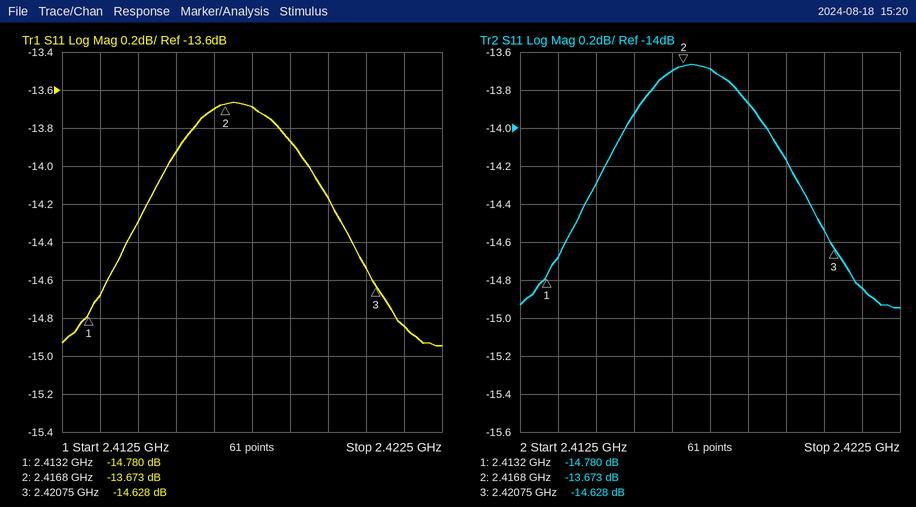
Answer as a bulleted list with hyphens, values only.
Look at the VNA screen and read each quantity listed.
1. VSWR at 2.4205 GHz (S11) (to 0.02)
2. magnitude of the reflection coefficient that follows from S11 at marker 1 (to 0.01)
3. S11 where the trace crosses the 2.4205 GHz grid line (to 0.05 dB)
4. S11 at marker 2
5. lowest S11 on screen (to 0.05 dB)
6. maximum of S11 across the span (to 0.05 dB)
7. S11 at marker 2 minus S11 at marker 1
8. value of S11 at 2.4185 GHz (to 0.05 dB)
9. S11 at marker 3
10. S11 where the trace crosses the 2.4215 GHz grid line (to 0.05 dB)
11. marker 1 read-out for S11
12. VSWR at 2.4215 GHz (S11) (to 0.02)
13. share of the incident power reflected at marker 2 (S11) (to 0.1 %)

- 1.46
- 0.18
- -14.55 dB
- -13.673 dB
- -14.95 dB
- -13.65 dB
- 1.107 dB
- -13.85 dB
- -14.628 dB
- -14.85 dB
- -14.780 dB
- 1.44
- 4.3 %
